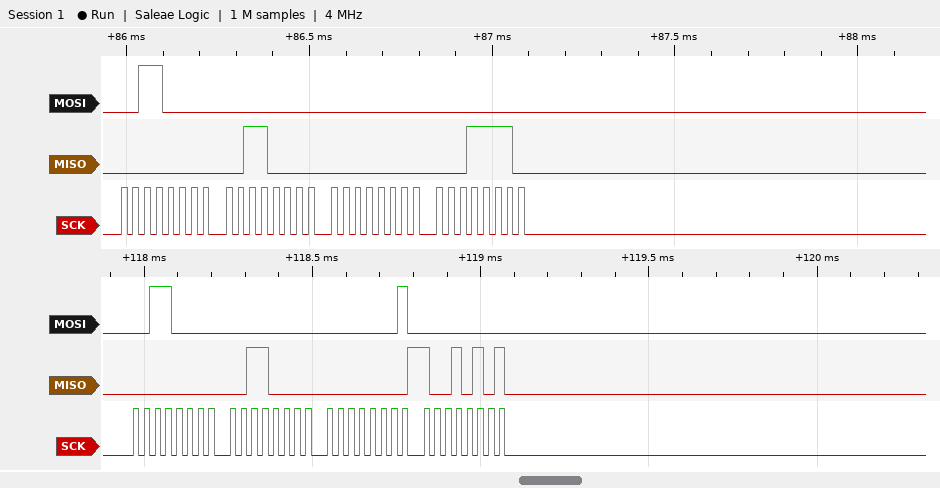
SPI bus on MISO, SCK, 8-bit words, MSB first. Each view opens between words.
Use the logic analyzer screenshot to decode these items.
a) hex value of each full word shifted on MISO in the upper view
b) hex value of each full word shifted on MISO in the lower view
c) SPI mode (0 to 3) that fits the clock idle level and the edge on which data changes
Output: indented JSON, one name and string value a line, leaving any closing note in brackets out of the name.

{
  "hex value of each full word shifted on MISO in the upper view": "00, 30, 00, 1E",
  "hex value of each full word shifted on MISO in the lower view": "00, 30, 00, 95",
  "SPI mode (0 to 3) that fits the clock idle level and the edge on which data changes": "0"
}
